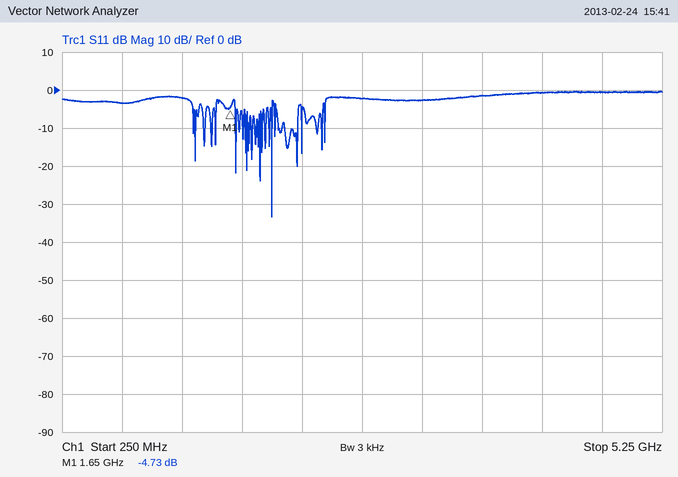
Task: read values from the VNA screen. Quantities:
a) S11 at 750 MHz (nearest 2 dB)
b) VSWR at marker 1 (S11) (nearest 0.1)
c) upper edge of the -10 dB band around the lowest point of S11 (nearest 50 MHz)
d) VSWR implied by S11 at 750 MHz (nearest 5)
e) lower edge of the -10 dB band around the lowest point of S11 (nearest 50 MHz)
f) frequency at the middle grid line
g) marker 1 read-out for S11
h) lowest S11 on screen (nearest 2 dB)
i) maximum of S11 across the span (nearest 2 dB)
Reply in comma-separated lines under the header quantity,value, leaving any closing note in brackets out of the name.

quantity,value
S11 at 750 MHz,-4 dB
VSWR at marker 1 (S11),3.8
upper edge of the -10 dB band around the lowest point of S11,2.00 GHz
VSWR implied by S11 at 750 MHz,5
lower edge of the -10 dB band around the lowest point of S11,2.00 GHz
frequency at the middle grid line,2.75 GHz
marker 1 read-out for S11,-4.73 dB
lowest S11 on screen,-34 dB
maximum of S11 across the span,0 dB
